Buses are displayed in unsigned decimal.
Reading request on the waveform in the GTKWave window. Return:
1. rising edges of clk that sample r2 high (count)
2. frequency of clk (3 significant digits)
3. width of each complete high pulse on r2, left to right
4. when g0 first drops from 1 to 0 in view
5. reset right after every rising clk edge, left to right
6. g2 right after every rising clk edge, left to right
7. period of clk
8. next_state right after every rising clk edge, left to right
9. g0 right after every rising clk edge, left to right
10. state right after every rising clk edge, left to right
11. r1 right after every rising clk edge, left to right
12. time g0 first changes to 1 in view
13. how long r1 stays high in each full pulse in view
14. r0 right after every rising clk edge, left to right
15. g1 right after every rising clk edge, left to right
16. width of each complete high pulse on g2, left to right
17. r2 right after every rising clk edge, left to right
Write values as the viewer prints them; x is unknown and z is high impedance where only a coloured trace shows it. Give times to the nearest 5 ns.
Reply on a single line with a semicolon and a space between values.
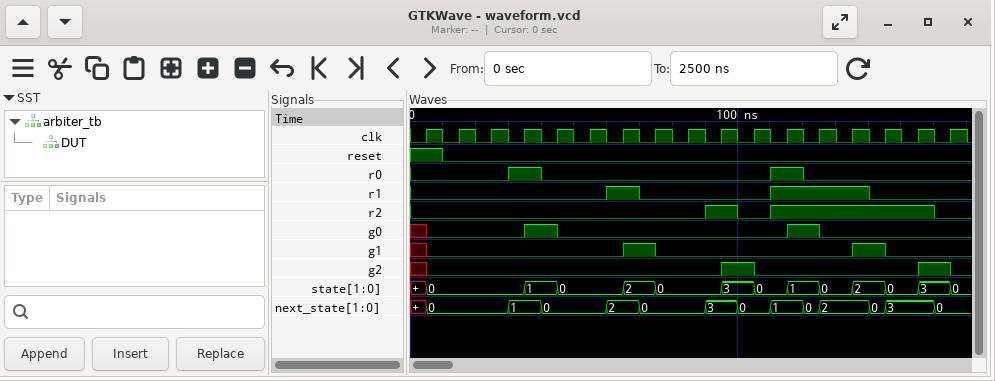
6; 100 MHz; 10 ns, 50 ns; 45 ns; 1 0 0 0 0 0 0 0 0 0 0 0 0 0 0 0 0; 0 0 0 0 0 0 0 0 0 1 0 0 0 0 0 1 0; 10 ns; 0, 0, 0, 1, 0, 0, 2, 0, 0, 3, 0, 1, 2, 2, 3, 3, 0; 0 0 0 1 0 0 0 0 0 0 0 1 0 0 0 0 0; 0, 0, 0, 1, 0, 0, 2, 0, 0, 3, 0, 1, 0, 2, 0, 3, 0; 0 0 0 0 0 0 1 0 0 0 0 1 1 1 0 0 0; 35 ns; 10 ns, 30 ns; 0 0 0 1 0 0 0 0 0 0 0 1 0 0 0 0 0; 0 0 0 0 0 0 1 0 0 0 0 0 0 1 0 0 0; 10 ns, 10 ns; 0 0 0 0 0 0 0 0 0 1 0 1 1 1 1 1 0
